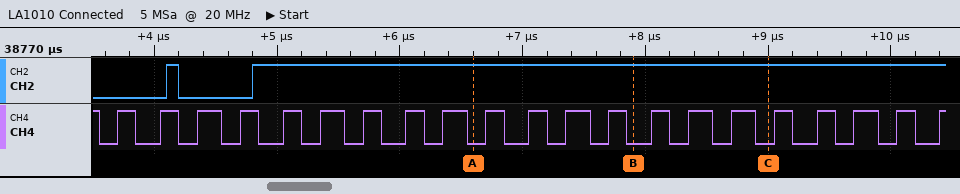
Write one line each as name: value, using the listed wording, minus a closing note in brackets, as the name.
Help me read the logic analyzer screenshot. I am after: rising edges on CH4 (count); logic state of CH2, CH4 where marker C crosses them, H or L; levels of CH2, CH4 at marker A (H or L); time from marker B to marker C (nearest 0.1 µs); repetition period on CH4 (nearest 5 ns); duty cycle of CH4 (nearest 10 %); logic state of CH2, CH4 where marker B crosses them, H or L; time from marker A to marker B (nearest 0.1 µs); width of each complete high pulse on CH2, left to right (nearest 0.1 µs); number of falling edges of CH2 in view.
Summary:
rising edges on CH4: 21
logic state of CH2, CH4 where marker C crosses them, H or L: CH2=H, CH4=L
levels of CH2, CH4 at marker A: CH2=H, CH4=L
time from marker B to marker C: 1.1 µs
repetition period on CH4: 335 ns
duty cycle of CH4: 50 %
logic state of CH2, CH4 where marker B crosses them, H or L: CH2=H, CH4=L
time from marker A to marker B: 1.3 µs
width of each complete high pulse on CH2, left to right: 0.1 µs
number of falling edges of CH2 in view: 1
